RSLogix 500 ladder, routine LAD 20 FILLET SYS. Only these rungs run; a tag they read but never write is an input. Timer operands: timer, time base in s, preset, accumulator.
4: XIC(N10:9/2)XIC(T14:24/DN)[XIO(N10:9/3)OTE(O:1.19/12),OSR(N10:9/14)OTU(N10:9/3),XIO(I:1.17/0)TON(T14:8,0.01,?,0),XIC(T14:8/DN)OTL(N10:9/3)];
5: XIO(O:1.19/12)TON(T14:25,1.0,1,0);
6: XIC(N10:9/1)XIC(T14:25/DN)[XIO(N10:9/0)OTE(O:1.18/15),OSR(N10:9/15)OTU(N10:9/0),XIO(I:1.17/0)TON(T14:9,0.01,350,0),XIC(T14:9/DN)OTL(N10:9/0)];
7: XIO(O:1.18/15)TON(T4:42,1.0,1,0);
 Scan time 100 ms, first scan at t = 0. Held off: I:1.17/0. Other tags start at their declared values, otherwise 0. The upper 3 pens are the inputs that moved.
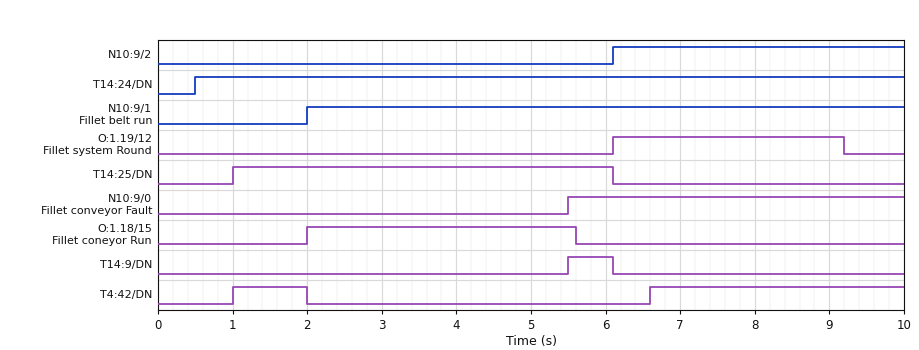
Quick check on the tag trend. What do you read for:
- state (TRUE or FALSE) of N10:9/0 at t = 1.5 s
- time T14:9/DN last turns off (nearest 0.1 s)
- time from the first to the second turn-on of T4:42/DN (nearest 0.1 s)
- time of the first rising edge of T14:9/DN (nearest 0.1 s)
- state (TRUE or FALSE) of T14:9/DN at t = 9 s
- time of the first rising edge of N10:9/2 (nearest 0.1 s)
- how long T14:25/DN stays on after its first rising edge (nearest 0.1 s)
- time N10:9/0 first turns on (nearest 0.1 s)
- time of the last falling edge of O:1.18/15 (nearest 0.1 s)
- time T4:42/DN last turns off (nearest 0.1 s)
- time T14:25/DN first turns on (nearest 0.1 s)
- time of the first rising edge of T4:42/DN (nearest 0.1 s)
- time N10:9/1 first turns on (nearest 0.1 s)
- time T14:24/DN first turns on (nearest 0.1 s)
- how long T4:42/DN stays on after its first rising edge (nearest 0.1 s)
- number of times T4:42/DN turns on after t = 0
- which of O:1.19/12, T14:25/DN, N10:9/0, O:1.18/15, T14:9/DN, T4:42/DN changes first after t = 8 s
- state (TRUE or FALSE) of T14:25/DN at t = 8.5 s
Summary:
FALSE
6.1 s
5.6 s
5.5 s
FALSE
6.1 s
5.1 s
5.5 s
5.6 s
2.0 s
1.0 s
1.0 s
2.0 s
0.5 s
1.0 s
2
O:1.19/12
FALSE
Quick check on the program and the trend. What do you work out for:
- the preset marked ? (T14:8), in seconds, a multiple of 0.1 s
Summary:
3.0 s
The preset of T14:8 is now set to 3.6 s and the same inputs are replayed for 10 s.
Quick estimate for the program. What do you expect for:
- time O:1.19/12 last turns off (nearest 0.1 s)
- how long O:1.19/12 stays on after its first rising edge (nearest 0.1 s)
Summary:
9.8 s
3.7 s
